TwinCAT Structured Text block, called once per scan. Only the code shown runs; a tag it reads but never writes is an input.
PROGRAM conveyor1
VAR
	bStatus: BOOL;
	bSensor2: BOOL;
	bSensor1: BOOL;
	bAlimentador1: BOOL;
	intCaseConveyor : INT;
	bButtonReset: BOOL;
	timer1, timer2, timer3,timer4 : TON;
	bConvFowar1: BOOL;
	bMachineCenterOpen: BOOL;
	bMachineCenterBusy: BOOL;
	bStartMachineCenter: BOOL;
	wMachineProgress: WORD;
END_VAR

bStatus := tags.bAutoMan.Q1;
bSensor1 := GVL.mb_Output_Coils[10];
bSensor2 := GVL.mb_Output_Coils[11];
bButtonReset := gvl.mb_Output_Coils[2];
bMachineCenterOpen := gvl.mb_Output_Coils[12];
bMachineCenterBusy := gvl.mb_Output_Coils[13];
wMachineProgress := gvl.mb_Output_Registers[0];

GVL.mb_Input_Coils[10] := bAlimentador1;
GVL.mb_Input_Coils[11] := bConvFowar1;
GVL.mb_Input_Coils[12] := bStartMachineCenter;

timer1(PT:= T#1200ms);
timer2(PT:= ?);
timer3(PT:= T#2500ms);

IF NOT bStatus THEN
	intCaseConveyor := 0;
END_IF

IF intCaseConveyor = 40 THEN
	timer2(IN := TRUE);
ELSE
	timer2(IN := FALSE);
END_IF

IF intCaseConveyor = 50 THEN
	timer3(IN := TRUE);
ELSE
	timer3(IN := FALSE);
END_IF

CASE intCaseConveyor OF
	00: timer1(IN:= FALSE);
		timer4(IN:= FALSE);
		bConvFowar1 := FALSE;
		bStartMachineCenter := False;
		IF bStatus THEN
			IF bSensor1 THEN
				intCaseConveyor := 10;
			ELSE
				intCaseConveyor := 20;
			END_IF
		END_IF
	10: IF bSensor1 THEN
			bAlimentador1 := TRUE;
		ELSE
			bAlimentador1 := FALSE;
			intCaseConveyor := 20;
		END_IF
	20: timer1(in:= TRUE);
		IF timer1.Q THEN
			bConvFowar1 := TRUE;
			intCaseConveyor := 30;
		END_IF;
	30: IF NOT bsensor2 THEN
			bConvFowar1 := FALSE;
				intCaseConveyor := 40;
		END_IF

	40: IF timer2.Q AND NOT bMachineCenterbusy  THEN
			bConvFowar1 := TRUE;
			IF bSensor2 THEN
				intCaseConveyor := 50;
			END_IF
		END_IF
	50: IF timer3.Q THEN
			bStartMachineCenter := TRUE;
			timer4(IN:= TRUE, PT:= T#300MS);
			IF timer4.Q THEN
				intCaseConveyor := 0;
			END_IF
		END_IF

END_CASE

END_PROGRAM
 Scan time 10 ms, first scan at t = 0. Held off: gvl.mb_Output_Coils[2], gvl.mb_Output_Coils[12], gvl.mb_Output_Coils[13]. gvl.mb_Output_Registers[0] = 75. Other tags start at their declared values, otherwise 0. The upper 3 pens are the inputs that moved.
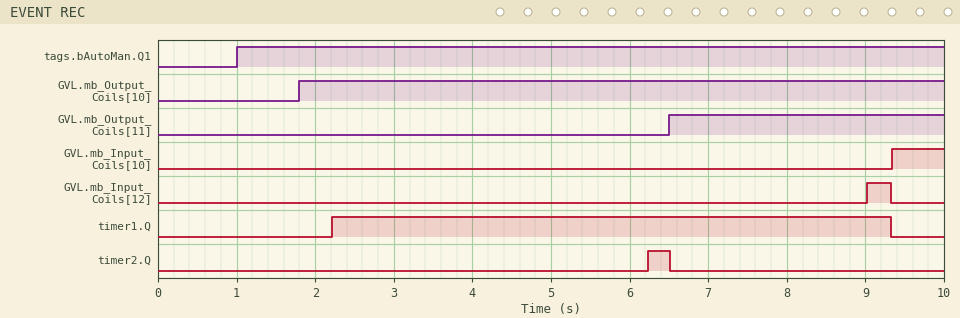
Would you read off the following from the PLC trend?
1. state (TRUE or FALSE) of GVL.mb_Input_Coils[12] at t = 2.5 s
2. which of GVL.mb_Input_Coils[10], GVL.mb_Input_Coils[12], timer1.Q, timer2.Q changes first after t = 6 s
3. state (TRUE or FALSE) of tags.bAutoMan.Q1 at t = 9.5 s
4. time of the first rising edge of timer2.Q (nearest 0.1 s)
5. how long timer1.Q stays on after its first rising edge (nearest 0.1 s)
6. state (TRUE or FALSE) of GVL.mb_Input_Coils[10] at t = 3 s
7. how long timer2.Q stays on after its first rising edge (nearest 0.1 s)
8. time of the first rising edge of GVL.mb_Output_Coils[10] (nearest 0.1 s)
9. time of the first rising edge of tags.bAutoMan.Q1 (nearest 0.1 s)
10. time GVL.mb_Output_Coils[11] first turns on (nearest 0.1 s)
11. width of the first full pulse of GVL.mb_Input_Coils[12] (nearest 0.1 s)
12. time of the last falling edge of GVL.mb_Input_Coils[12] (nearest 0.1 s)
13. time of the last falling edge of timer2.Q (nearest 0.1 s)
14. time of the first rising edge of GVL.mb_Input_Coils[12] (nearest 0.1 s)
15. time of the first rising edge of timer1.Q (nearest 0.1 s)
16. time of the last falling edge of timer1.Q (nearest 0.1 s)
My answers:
FALSE
timer2.Q
TRUE
6.2 s
7.1 s
FALSE
0.3 s
1.8 s
1.0 s
6.5 s
0.3 s
9.3 s
6.5 s
9.0 s
2.2 s
9.3 s
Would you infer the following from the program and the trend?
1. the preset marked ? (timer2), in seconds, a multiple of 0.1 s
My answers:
4.0 s
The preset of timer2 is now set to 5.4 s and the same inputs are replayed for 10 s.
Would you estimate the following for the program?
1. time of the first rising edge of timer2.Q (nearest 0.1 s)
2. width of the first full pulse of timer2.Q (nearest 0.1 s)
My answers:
7.6 s
0.0 s
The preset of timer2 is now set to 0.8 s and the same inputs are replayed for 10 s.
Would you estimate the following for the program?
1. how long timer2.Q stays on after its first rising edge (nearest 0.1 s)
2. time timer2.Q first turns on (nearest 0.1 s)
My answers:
3.5 s
3.0 s
